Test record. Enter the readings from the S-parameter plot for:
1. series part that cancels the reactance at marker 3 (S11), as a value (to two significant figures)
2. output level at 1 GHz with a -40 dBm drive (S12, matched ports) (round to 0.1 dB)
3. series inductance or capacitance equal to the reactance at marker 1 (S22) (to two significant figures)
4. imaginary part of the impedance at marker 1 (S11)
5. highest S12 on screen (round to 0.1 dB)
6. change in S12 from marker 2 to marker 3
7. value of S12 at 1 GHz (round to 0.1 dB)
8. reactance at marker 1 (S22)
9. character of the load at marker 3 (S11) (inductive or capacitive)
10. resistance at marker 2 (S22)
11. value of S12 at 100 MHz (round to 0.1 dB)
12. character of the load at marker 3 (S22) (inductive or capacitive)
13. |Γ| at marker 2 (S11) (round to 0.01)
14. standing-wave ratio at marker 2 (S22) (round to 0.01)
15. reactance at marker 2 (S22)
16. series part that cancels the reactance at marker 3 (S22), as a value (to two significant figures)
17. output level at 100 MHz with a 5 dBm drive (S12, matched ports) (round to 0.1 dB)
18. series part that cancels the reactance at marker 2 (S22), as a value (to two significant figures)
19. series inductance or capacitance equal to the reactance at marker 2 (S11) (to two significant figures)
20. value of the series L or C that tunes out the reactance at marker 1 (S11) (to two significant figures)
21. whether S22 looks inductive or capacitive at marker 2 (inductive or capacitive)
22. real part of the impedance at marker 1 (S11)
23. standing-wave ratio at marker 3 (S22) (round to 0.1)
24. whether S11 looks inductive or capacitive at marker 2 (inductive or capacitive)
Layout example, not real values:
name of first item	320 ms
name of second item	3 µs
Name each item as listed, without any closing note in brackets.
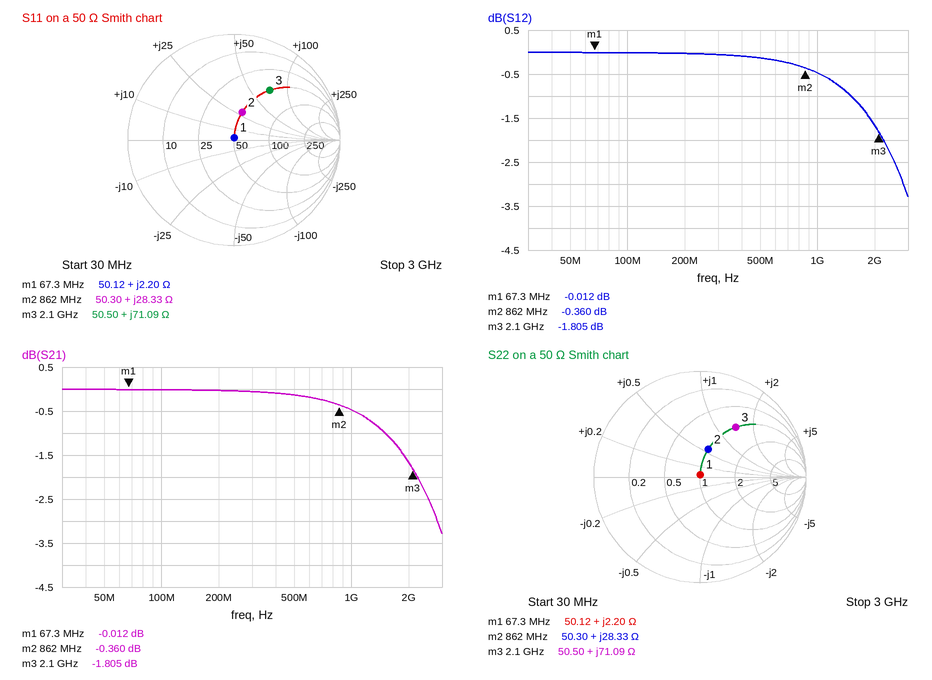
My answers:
series part that cancels the reactance at marker 3 (S11), as a value	1.1 pF
output level at 1 GHz with a -40 dBm drive (S12, matched ports)	-40.5 dBm
series inductance or capacitance equal to the reactance at marker 1 (S22)	5.2 nH
imaginary part of the impedance at marker 1	+2.20 Ω
highest S12 on screen	0.0 dB
change in S12 from marker 2 to marker 3	-1.445 dB
value of S12 at 1 GHz	-0.5 dB
reactance at marker 1	+2.20 Ω
character of the load at marker 3 (S11)	inductive
resistance at marker 2	50.30 Ω
value of S12 at 100 MHz	0.0 dB
character of the load at marker 3 (S22)	inductive
|Γ| at marker 2 (S11)	0.27
standing-wave ratio at marker 2 (S22)	1.75
reactance at marker 2	+28.33 Ω
series part that cancels the reactance at marker 3 (S22), as a value	1.1 pF
output level at 100 MHz with a 5 dBm drive (S12, matched ports)	5.0 dBm
series part that cancels the reactance at marker 2 (S22), as a value	6.5 pF
series inductance or capacitance equal to the reactance at marker 2 (S11)	5.2 nH
value of the series L or C that tunes out the reactance at marker 1 (S11)	1.1 nF
whether S22 looks inductive or capacitive at marker 2	inductive
real part of the impedance at marker 1	50.12 Ω
standing-wave ratio at marker 3 (S22)	3.7
whether S11 looks inductive or capacitive at marker 2	inductive
